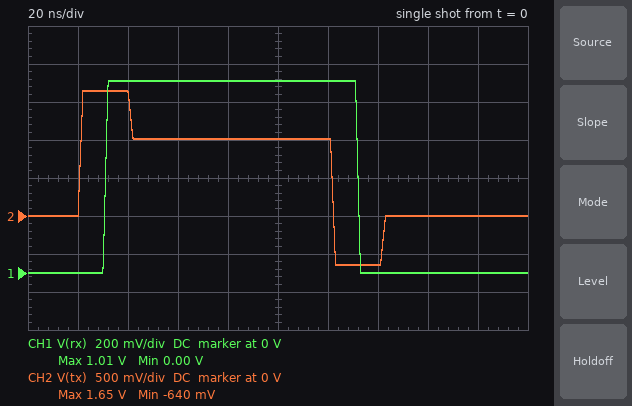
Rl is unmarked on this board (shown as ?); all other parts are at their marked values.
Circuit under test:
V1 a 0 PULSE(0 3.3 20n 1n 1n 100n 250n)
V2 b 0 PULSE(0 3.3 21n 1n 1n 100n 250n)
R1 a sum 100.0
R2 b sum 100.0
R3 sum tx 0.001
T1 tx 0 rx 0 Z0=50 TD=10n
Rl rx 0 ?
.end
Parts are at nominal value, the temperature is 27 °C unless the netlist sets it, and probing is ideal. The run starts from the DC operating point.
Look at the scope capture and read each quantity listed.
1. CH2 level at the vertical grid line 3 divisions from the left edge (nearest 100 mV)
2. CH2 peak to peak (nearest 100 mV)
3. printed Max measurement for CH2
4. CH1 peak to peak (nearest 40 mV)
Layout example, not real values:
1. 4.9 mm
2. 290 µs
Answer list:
1. 1.0 V
2. 2.3 V
3. 1.65 V
4. 1.00 V
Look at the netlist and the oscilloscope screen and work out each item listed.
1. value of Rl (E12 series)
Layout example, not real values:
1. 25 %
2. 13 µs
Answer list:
1. 22 Ω
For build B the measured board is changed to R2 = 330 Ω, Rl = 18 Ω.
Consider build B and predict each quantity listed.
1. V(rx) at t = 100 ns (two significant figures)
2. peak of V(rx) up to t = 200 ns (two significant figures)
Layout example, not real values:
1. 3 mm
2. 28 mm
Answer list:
1. 630 mV
2. 690 mV
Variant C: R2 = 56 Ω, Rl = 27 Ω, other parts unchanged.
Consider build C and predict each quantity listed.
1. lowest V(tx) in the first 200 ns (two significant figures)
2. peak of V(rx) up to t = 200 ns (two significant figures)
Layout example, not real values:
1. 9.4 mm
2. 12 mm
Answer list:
1. -500 mV
2. 1.4 V
